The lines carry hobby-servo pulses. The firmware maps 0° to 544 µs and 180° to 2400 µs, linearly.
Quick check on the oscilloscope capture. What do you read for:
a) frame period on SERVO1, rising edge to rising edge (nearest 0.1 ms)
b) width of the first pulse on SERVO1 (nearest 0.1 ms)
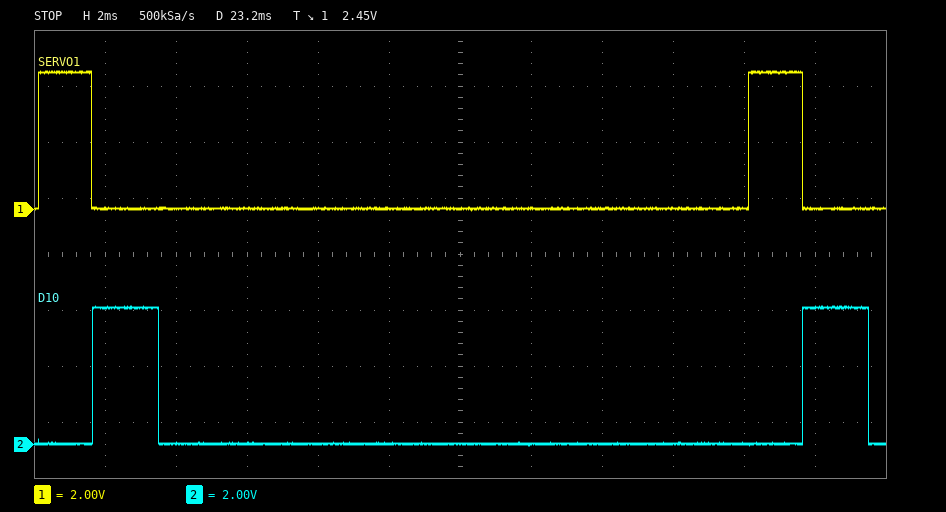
20.0 ms
1.5 ms
